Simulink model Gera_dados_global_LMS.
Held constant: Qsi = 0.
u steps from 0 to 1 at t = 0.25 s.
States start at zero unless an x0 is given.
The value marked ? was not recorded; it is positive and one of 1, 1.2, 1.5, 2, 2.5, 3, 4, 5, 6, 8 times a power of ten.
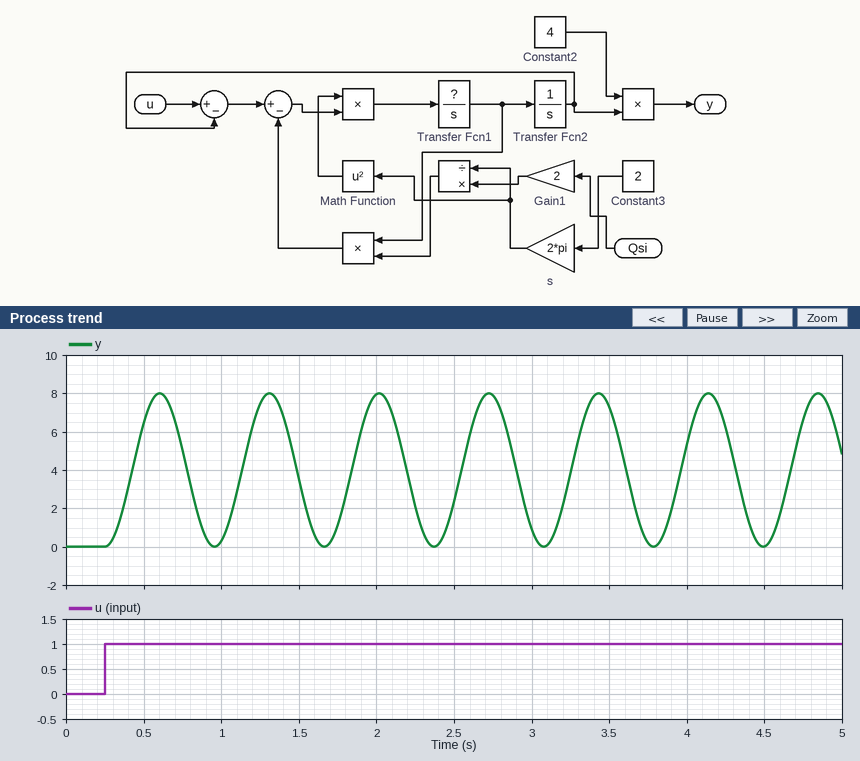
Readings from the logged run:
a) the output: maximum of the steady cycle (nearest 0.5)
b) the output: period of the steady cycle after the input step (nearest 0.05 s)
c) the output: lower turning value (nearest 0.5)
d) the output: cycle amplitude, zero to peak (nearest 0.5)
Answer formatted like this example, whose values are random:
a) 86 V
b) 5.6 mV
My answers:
a) 8.0
b) 0.70 s
c) 0.0
d) 4.0
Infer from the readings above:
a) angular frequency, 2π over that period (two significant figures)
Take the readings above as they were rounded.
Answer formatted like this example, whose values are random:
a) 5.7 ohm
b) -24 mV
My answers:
a) 9.0 rad/s
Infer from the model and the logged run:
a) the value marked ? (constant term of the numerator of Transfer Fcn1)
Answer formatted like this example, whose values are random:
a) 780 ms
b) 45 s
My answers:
a) 0.5
